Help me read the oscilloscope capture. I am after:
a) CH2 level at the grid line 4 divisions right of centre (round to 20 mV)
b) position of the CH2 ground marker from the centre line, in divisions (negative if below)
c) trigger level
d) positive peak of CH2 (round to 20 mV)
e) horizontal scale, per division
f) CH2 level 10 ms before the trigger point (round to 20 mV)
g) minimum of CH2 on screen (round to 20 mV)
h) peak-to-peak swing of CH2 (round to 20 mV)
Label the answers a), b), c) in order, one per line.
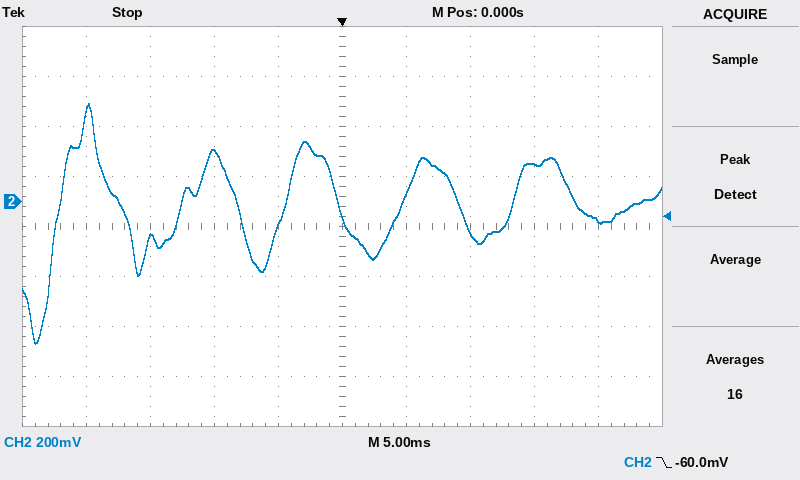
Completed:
a) -80 mV
b) +0.5 div
c) -60.0 mV
d) 400 mV
e) 5 ms
f) 200 mV
g) -560 mV
h) 960 mV
